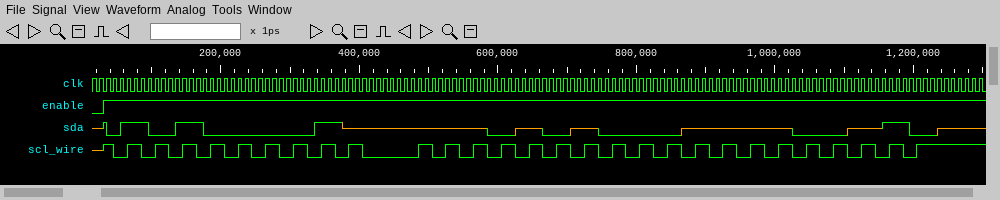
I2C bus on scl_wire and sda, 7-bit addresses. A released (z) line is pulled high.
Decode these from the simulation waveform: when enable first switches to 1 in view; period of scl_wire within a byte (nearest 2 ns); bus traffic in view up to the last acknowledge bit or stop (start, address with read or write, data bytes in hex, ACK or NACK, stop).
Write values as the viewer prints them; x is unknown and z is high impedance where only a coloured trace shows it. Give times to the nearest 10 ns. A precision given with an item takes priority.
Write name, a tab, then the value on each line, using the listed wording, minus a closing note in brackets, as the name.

when enable first switches to 1 in view	30 ns
period of scl_wire within a byte	40 ns
bus traffic in view up to the last acknowledge bit or stop	start, address 50 read NACK, EA ACK, 79 NACK, stop
